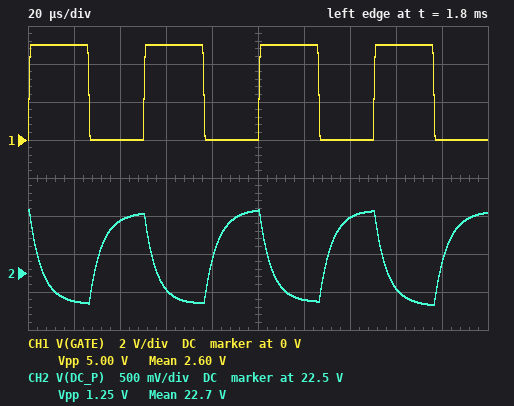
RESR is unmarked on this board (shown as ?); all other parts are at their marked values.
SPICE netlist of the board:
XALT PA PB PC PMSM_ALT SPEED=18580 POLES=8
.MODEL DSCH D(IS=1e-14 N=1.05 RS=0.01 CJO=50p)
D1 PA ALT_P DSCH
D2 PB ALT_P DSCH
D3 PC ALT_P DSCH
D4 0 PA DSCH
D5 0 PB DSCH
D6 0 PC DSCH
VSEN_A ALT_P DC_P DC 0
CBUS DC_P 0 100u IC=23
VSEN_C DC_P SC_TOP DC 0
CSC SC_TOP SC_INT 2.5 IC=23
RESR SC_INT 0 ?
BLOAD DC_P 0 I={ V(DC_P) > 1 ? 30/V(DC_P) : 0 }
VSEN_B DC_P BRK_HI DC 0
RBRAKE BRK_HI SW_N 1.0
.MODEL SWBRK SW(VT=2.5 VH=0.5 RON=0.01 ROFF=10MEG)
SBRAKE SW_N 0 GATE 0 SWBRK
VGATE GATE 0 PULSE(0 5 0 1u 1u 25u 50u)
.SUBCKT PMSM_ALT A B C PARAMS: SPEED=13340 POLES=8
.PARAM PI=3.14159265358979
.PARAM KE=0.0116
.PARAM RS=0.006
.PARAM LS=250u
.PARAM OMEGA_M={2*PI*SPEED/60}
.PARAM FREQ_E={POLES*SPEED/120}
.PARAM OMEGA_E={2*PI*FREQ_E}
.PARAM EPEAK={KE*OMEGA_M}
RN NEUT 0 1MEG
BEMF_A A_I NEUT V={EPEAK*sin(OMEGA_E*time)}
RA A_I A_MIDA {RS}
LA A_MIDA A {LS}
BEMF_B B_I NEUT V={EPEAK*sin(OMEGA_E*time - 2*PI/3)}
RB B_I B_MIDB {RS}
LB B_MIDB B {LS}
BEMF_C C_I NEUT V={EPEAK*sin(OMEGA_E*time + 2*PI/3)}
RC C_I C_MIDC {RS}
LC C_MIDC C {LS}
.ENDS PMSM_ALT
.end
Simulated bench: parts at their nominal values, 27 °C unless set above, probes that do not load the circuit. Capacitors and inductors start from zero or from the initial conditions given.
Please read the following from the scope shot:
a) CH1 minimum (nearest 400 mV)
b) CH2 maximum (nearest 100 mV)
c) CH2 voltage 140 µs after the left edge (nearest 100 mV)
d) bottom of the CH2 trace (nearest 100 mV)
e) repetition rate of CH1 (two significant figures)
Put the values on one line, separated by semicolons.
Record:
0 V; 23.3 V; 23.2 V; 22.1 V; 20 kHz
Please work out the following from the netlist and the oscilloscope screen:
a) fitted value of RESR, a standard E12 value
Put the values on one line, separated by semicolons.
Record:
0.056 Ω
